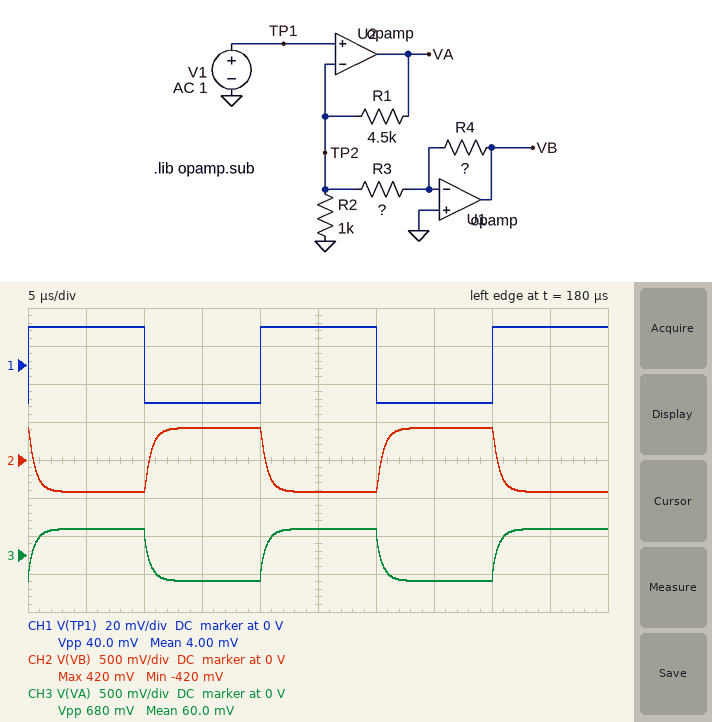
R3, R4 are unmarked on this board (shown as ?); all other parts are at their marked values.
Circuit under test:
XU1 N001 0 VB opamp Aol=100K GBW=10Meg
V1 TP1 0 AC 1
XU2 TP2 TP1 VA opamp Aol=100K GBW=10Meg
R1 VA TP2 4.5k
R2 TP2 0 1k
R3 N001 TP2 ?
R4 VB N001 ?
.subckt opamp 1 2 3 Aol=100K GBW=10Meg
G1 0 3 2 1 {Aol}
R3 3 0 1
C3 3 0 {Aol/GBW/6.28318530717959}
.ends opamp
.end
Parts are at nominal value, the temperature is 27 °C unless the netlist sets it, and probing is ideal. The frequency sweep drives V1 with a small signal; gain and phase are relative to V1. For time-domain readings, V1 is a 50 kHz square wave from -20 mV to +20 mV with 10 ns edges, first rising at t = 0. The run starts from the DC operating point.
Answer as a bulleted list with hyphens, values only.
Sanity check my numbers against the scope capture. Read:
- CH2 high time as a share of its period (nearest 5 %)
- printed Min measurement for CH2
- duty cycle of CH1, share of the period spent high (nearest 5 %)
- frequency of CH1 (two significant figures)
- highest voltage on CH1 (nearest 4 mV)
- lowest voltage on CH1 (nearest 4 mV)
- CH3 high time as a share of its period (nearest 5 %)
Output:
- 50 %
- -420 mV
- 50 %
- 50 kHz
- 20 mV
- -20 mV
- 50 %
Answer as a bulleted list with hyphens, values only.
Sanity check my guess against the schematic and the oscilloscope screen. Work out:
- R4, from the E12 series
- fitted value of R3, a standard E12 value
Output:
- 8.2 kΩ
- 390 Ω
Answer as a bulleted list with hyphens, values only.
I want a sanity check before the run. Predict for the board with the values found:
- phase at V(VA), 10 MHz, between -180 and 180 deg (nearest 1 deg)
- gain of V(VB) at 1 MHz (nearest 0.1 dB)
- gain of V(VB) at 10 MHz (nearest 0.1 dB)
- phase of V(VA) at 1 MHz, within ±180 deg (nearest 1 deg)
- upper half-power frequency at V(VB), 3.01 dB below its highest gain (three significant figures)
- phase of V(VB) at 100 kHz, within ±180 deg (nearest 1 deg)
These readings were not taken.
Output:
- -81 deg
- 14.6 dB
- -16.3 dB
- -57 deg
- 280 kHz
- 158 deg
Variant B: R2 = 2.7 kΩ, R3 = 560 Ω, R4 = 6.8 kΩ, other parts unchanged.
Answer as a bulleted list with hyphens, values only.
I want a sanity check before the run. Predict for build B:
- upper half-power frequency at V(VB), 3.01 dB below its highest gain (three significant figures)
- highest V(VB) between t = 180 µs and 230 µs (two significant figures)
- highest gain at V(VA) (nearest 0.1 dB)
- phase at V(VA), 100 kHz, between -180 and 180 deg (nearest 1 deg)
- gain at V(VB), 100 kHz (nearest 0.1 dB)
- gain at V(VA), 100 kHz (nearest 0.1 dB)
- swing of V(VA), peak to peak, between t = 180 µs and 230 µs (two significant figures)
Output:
- 454 kHz
- 240 mV
- 20.6 dB
- -11 deg
- 21.5 dB
- 20.4 dB
- 430 mV
